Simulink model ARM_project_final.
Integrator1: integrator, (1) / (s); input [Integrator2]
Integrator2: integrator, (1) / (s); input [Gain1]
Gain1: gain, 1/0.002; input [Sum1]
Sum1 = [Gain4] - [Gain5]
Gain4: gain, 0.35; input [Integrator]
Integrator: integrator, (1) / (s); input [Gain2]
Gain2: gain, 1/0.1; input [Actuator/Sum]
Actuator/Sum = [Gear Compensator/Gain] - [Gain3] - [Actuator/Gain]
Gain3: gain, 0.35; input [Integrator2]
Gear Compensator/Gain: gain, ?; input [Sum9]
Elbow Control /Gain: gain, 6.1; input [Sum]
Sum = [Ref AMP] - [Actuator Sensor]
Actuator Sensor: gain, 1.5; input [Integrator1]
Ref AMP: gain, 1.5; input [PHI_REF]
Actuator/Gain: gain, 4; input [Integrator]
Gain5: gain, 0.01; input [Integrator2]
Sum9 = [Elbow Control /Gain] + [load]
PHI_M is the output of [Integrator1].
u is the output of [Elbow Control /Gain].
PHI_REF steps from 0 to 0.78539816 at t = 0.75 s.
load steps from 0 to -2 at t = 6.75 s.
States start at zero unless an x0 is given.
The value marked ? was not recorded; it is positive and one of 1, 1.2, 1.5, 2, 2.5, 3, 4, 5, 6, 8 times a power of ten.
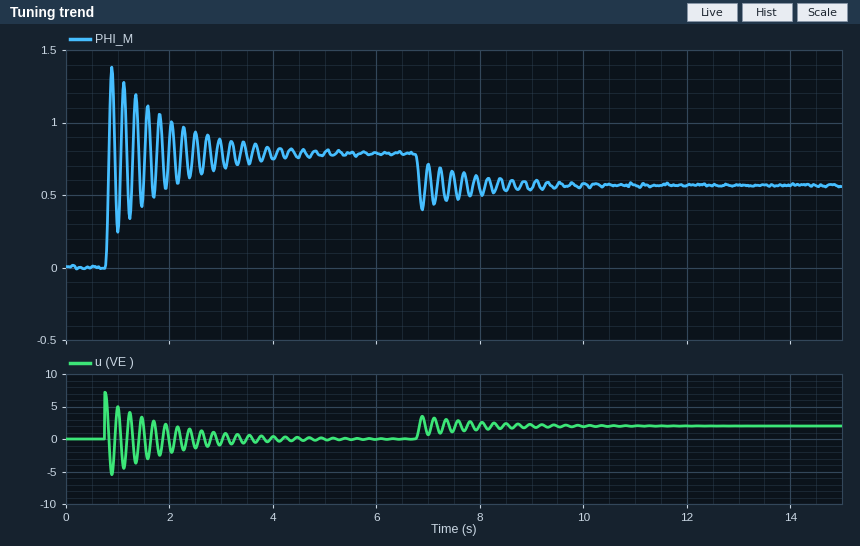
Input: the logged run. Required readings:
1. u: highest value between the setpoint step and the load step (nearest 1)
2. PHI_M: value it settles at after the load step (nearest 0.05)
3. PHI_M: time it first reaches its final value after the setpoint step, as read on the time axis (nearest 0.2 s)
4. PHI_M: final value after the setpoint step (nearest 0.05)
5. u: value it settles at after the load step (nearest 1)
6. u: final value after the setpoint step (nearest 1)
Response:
7
0.55
0.8 s
0.80
2
0
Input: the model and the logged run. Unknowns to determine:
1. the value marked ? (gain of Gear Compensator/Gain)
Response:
2
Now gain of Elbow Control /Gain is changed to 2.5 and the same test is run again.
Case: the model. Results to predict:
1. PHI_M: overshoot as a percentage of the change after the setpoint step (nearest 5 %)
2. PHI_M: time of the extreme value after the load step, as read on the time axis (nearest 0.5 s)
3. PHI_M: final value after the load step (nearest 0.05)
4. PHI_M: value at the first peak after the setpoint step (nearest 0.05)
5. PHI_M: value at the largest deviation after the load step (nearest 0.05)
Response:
30 %
7.0 s
0.25
1.00
0.10
